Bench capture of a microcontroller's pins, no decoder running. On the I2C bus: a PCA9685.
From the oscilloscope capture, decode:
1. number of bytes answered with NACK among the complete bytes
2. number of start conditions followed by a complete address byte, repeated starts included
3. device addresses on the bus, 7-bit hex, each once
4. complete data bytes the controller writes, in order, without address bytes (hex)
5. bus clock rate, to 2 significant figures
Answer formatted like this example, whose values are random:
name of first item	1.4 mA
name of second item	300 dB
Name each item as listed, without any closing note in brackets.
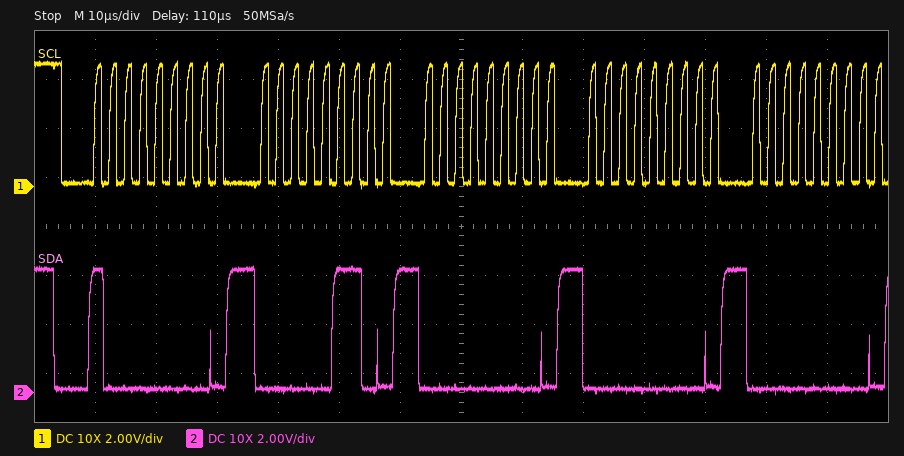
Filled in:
number of bytes answered with NACK among the complete bytes	0
number of start conditions followed by a complete address byte, repeated starts included	1
device addresses on the bus, 7-bit hex, each once	0x40
complete data bytes the controller writes, in order, without address bytes	06 00 00 00
bus clock rate, to 2 significant figures	400 kHz
